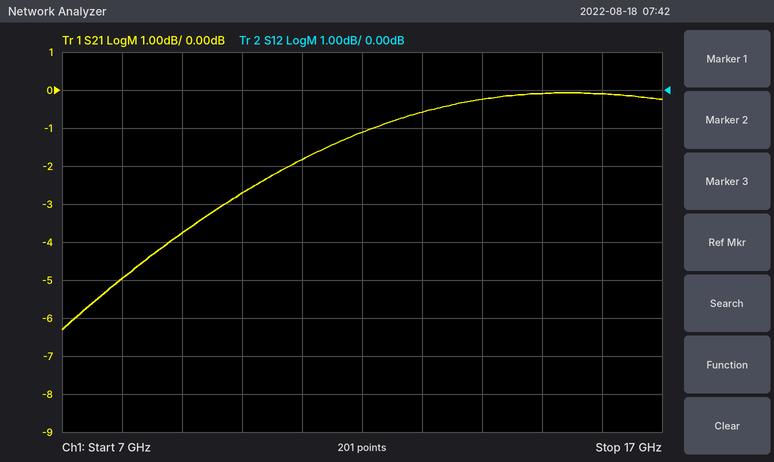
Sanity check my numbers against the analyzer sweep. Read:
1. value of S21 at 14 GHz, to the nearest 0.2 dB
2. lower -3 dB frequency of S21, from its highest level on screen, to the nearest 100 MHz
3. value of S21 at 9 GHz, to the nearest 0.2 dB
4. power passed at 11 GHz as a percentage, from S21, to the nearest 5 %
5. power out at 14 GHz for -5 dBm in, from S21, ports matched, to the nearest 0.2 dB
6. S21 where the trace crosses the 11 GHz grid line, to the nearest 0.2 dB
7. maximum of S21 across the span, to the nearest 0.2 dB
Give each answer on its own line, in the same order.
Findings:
-0.2 dB
9.6 GHz
-3.8 dB
65 %
-5.2 dBm
-1.8 dB
0.0 dB
